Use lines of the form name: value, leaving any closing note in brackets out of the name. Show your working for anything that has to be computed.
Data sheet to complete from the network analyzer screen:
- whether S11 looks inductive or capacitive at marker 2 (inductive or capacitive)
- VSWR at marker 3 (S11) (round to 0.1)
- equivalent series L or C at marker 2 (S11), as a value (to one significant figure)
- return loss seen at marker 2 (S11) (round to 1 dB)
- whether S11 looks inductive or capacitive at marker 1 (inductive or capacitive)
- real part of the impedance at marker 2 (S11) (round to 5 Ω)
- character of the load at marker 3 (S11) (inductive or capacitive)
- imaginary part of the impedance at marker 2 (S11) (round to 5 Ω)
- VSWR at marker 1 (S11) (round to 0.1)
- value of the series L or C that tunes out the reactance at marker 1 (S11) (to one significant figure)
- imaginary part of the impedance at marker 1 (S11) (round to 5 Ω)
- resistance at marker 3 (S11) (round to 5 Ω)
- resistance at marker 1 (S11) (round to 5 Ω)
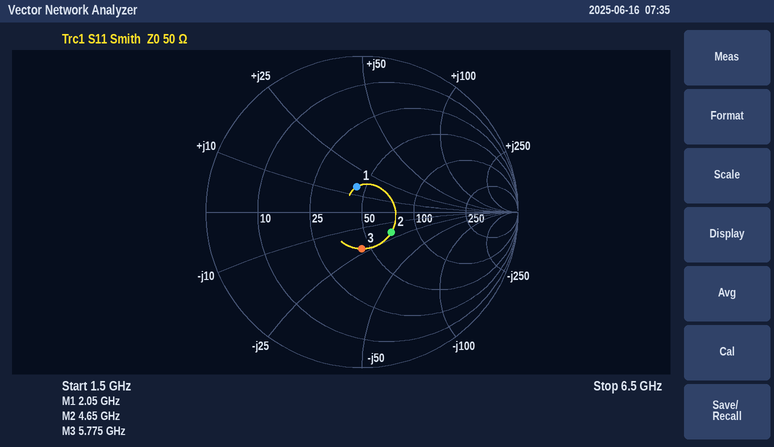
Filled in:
whether S11 looks inductive or capacitive at marker 2: capacitive
VSWR at marker 3 (S11): 1.6
equivalent series L or C at marker 2 (S11), as a value: C = 1/(2π × 4.65 GHz × 20 Ω) ≈ 2 pF
return loss seen at marker 2 (S11): 13 dB
whether S11 looks inductive or capacitive at marker 1: inductive
real part of the impedance at marker 2 (S11): 70 Ω
character of the load at marker 3 (S11): capacitive
imaginary part of the impedance at marker 2 (S11): -20 Ω
VSWR at marker 1 (S11): 1.4
value of the series L or C that tunes out the reactance at marker 1 (S11): C = 1/(2π × 2.05 GHz × 15 Ω) ≈ 5 pF
imaginary part of the impedance at marker 1 (S11): +15 Ω
resistance at marker 3 (S11): 45 Ω
resistance at marker 1 (S11): 45 Ω
